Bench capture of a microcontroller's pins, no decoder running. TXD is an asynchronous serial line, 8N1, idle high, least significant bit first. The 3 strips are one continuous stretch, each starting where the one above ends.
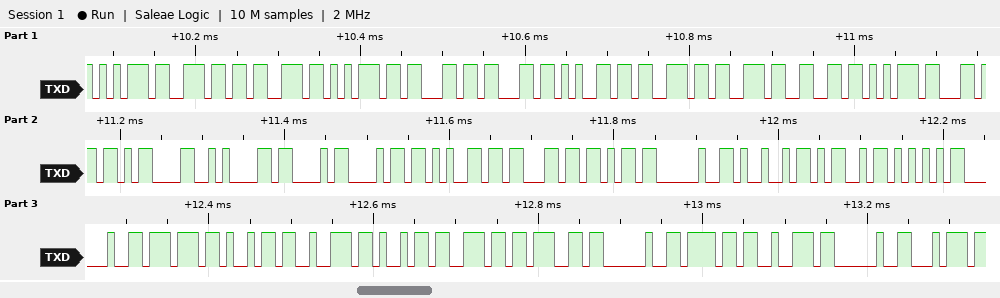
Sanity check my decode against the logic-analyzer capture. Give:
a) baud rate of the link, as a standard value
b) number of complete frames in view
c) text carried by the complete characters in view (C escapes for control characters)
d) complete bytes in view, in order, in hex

115200 baud
35
"unsuccessful\r\nCheck IMU wiring or t"
75 6E 73 75 63 63 65 73 73 66 75 6C 0D 0A 43 68 65 63 6B 20 49 4D 55 20 77 69 72 69 6E 67 20 6F 72 20 74
